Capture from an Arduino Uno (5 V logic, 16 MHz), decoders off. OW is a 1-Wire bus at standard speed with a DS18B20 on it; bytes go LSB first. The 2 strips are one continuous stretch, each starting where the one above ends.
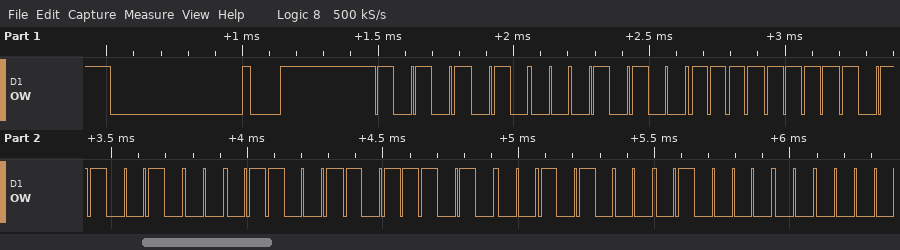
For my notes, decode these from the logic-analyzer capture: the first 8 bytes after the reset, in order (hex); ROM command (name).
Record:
55 28 FF 4D 98 5D 14 02
Match ROM
